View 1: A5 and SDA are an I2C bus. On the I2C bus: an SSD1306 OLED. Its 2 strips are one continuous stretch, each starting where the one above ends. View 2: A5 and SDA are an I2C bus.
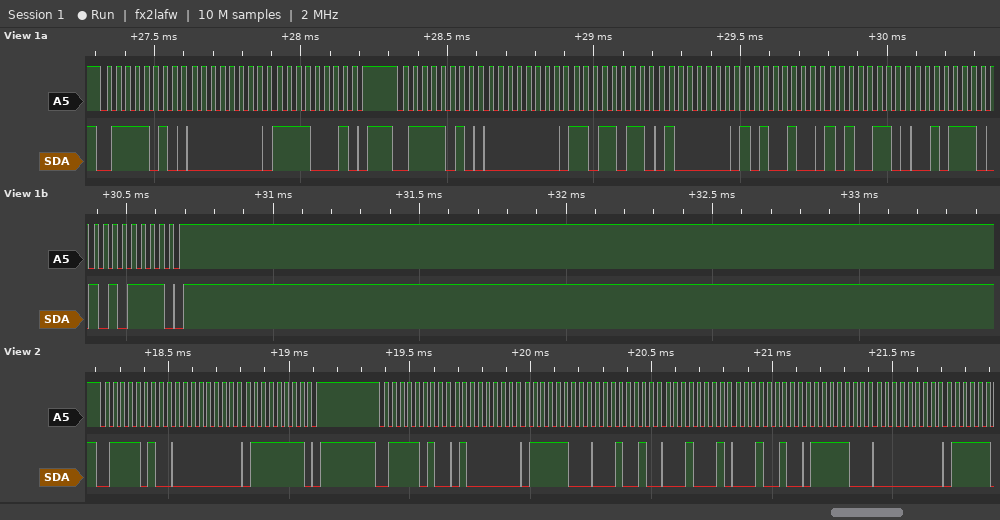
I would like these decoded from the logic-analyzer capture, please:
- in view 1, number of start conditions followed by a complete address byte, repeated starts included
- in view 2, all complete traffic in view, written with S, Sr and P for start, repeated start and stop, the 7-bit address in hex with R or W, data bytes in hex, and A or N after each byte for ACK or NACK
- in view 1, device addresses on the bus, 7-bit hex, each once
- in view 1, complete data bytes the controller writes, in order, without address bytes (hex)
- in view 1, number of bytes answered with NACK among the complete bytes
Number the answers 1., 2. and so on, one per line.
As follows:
1. 2
2. S 3DW A 00 A 7F A P S 3DW A 40 A 7C A 12 A 11 A 12 A 7C A 00 A
3. 0x3D
4. 00 F1 00 DB 40 A4 A6 2E AF
5. 0
